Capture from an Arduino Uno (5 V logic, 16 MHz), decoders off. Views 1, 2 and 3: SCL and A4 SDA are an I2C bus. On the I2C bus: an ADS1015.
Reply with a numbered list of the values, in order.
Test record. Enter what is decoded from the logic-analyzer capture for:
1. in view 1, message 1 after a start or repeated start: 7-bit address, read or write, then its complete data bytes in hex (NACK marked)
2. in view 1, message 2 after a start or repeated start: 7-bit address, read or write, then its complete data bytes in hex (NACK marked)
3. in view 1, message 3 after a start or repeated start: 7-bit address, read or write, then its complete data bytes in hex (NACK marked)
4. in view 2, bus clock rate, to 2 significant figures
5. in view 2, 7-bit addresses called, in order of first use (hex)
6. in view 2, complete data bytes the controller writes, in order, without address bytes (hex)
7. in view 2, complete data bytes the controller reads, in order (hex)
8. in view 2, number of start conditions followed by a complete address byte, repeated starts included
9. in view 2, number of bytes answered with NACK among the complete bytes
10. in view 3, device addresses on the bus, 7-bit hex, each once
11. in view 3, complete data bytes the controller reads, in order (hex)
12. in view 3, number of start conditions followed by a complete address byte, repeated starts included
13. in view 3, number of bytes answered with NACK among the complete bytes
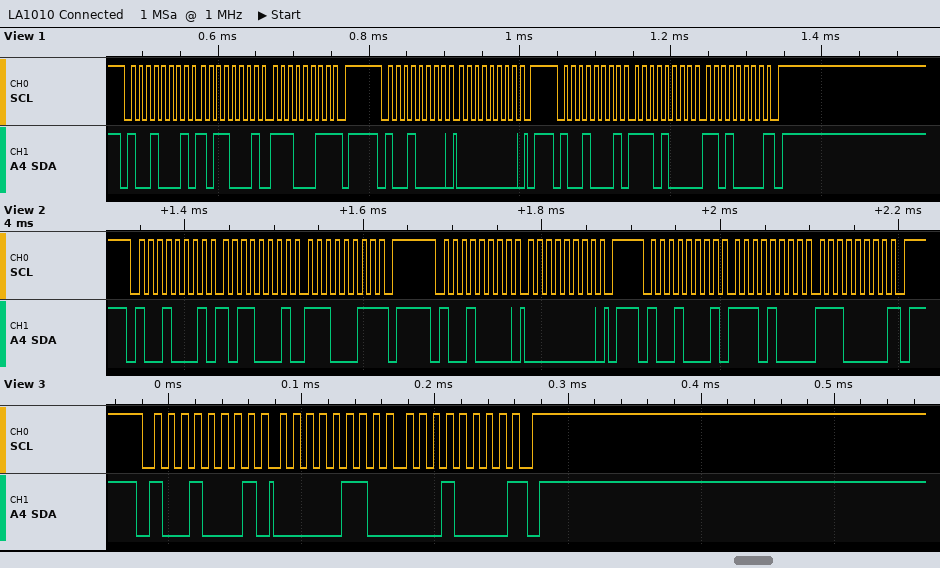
1. 0x48 read: B1 E3 NACK
2. 0x48 write: 00
3. 0x48 read: E8 D0 NACK
4. 100 kHz
5. 0x48
6. 00
7. B1 E3 E8 E0
8. 3
9. 2
10. 0x48
11. 06 10
12. 1
13. 1
